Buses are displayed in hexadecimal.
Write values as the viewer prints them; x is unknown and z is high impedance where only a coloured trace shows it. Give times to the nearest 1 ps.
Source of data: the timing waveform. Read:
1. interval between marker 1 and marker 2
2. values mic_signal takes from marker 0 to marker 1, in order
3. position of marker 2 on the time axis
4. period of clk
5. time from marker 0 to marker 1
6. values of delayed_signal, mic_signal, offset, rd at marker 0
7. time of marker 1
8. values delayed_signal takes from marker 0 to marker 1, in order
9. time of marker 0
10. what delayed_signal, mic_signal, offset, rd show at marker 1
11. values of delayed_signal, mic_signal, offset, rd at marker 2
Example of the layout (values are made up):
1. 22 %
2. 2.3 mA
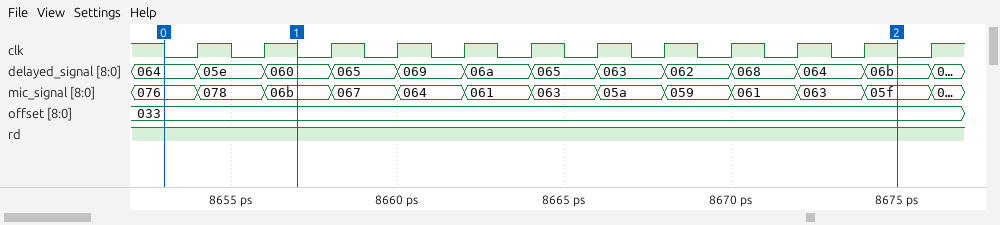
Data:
1. 18 ps
2. 076, 078, 06b
3. 8675 ps
4. 2 ps
5. 4 ps
6. delayed_signal=064, mic_signal=076, offset=033, rd=1
7. 8657 ps
8. 064, 05e, 060
9. 8653 ps
10. delayed_signal=060, mic_signal=06b, offset=033, rd=1
11. delayed_signal=06b, mic_signal=05f, offset=033, rd=1
